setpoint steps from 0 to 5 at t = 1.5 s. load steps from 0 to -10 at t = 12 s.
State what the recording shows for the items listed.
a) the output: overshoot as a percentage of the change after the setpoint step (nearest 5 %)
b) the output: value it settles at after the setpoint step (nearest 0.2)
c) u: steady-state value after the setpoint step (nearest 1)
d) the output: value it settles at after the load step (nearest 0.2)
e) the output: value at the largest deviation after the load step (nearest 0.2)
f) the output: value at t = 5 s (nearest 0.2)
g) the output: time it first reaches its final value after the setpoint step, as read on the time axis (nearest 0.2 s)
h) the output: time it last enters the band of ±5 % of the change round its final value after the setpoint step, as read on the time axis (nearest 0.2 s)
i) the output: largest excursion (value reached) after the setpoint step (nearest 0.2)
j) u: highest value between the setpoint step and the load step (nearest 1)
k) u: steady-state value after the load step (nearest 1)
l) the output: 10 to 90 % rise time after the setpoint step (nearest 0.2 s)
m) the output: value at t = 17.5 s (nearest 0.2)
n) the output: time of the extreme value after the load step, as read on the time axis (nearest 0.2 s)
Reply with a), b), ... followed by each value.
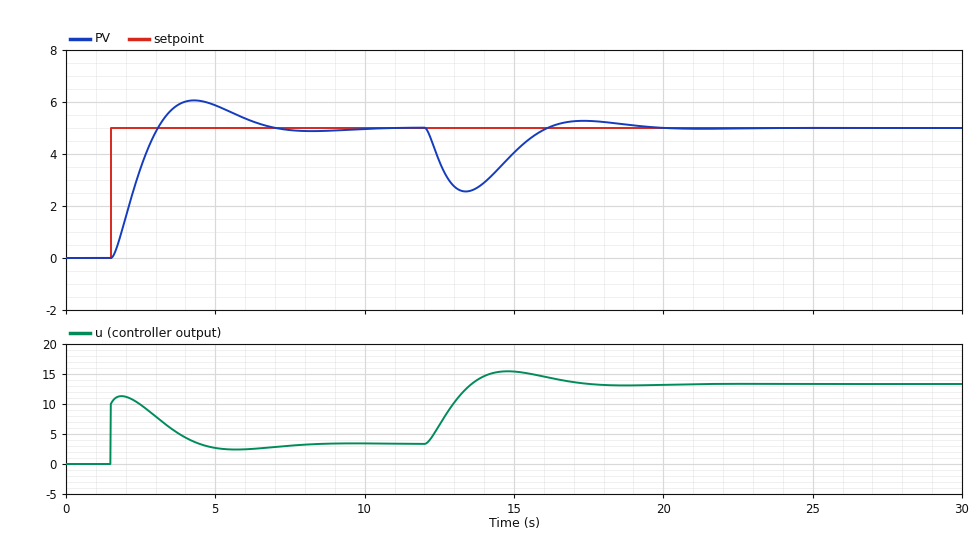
a) 20 %
b) 5.0
c) 3
d) 5.0
e) 2.6
f) 5.8
g) 3.0 s
h) 6.2 s
i) 6.0
j) 11
k) 13
l) 1.2 s
m) 5.2
n) 13.4 s
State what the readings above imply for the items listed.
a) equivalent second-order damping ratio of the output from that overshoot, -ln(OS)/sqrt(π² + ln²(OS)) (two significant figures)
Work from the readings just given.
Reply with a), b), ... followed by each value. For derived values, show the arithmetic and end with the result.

a) ln(0.2) = -1.609; 1.609 / sqrt(9.870 + 2.590) = 0.46
